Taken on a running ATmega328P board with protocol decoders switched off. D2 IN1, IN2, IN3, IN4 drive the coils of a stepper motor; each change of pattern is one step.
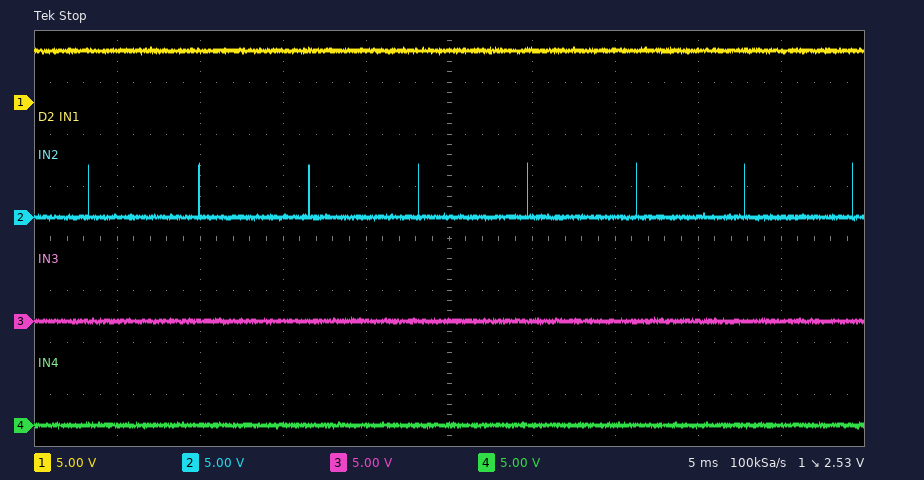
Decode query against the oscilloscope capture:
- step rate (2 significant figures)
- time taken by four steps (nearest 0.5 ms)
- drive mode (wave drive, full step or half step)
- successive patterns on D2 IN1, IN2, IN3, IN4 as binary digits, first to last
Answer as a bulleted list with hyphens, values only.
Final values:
- 150 steps/s
- 26.5 ms
- wave drive
- 1000 1000 1000 1000 1000 1000 1000 1000 1000
